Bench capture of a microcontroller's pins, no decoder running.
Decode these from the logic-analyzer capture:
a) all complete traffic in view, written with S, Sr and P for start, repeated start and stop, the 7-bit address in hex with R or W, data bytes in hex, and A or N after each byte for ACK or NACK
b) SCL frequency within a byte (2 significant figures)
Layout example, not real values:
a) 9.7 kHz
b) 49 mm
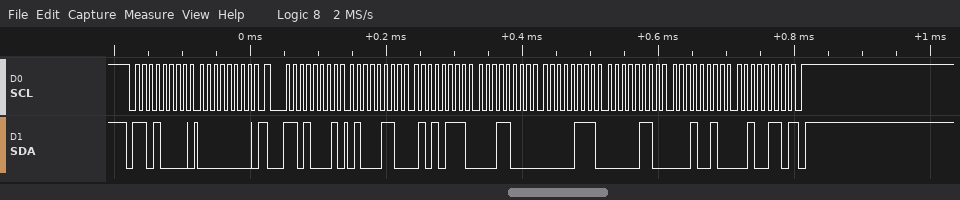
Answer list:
a) S 68W A 00 A Sr 68R A 46 A 57 A 18 A 07 A 06 A 12 A 26 N P
b) 100 kHz
